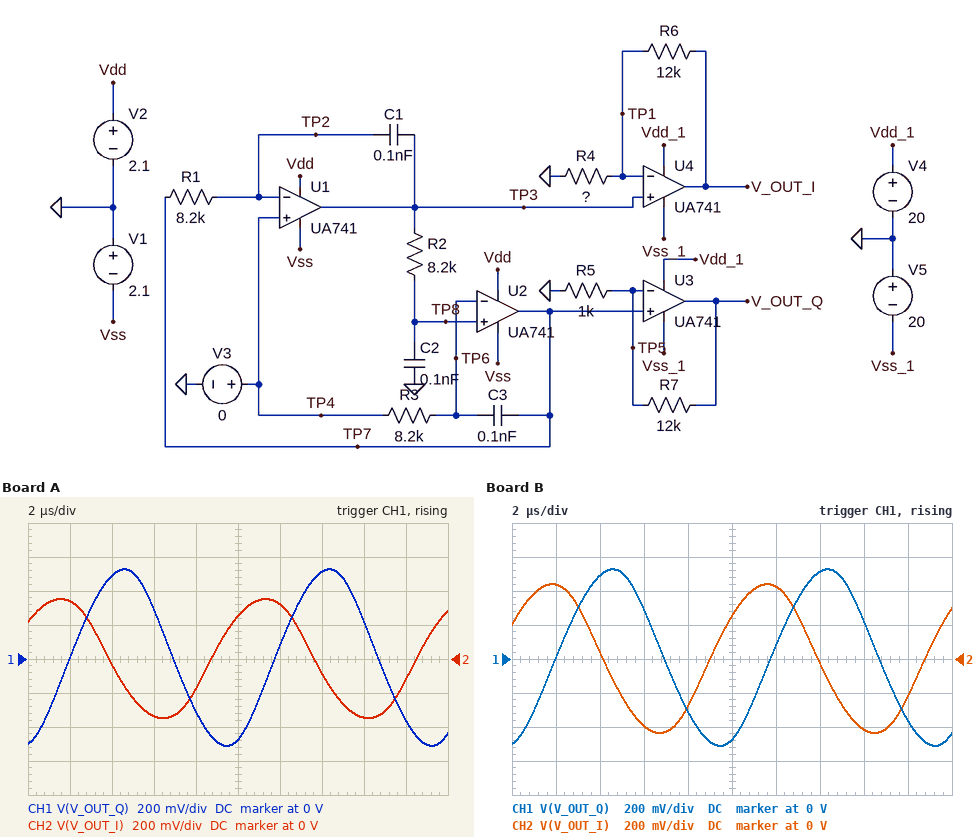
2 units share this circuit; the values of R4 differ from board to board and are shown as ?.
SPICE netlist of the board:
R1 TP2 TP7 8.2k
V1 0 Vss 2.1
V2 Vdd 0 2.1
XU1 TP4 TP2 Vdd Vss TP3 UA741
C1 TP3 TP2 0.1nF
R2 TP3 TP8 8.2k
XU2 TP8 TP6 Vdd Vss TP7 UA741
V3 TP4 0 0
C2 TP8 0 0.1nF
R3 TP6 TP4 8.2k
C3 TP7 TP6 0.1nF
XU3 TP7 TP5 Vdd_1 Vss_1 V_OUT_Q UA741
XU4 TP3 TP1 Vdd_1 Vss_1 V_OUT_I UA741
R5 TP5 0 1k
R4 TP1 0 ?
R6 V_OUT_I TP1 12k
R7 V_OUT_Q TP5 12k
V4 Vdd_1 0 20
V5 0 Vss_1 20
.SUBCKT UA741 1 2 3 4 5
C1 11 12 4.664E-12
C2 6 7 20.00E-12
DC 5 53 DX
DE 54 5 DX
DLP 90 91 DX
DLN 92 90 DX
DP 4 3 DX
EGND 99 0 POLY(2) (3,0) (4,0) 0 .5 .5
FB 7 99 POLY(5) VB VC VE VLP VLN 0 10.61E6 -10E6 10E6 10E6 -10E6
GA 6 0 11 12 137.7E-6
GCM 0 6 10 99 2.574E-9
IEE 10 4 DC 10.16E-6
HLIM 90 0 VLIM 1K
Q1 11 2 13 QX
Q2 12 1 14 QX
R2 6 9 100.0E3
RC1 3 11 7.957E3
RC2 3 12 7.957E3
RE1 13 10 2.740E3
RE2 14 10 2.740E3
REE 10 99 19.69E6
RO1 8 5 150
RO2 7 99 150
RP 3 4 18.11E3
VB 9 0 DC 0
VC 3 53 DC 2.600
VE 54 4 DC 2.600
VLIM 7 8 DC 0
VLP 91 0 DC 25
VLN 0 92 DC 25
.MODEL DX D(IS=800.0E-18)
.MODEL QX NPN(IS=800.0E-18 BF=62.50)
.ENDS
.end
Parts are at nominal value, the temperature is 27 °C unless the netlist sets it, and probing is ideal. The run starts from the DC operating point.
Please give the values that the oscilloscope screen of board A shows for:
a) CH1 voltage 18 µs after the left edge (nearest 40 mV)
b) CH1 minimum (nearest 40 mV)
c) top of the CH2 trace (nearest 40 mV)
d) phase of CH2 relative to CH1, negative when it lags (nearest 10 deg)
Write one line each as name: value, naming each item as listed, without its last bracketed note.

CH1 voltage 18 µs after the left edge: -360 mV
CH1 minimum: -520 mV
top of the CH2 trace: 360 mV
phase of CH2 relative to CH1, negative when it lags: 110 deg
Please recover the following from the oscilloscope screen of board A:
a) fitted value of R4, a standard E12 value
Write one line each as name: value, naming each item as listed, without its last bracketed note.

fitted value of R4, a standard E12 value: 2.2 kΩ
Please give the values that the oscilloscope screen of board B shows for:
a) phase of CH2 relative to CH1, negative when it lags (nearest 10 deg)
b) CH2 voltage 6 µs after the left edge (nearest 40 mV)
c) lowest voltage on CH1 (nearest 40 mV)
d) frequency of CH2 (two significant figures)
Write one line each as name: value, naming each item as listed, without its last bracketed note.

phase of CH2 relative to CH1, negative when it lags: 100 deg
CH2 voltage 6 µs after the left edge: -400 mV
lowest voltage on CH1: -520 mV
frequency of CH2: 100 kHz
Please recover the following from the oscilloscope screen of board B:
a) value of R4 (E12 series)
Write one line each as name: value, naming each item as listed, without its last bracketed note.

value of R4: 1.5 kΩ
